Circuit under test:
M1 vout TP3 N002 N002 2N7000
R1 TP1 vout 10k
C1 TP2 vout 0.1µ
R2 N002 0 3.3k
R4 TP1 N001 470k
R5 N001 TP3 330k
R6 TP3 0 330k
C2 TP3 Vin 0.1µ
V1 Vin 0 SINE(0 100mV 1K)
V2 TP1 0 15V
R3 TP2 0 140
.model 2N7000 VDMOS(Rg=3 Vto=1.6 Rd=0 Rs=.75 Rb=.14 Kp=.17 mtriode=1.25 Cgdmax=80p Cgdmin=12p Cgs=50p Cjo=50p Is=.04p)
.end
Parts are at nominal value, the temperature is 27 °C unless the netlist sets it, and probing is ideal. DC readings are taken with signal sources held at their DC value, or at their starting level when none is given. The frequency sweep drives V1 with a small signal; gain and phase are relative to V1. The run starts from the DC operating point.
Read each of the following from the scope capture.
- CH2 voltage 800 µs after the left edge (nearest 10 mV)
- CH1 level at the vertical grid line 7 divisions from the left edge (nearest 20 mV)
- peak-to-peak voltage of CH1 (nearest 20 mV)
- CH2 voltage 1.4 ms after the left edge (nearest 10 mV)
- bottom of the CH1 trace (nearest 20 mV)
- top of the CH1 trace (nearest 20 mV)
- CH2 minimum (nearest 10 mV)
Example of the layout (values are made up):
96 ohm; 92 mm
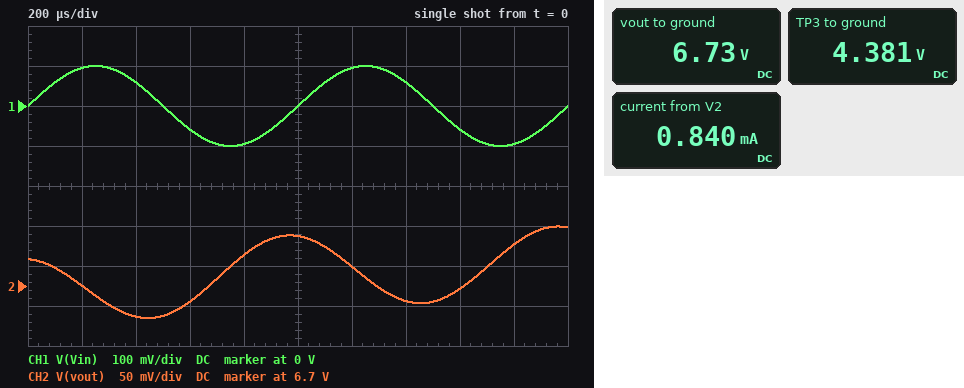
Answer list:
6.74 V; 60 mV; 200 mV; 6.68 V; -100 mV; 100 mV; 6.66 V
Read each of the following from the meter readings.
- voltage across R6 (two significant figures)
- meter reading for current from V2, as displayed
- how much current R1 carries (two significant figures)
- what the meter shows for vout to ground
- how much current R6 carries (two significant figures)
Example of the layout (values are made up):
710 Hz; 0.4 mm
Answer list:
4.4 V; 0.840 mA; 830 µA; 6.73 V; 13 µA
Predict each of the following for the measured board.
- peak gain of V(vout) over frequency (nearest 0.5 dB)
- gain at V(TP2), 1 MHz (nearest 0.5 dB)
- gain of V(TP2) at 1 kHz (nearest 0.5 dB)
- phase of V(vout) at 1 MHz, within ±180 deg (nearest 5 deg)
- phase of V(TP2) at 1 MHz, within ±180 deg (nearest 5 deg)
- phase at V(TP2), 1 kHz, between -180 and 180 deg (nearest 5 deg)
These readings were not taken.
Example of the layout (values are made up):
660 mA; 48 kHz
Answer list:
9.0 dB; -26.5 dB; -28.0 dB; 150 deg; 150 deg; -170 deg
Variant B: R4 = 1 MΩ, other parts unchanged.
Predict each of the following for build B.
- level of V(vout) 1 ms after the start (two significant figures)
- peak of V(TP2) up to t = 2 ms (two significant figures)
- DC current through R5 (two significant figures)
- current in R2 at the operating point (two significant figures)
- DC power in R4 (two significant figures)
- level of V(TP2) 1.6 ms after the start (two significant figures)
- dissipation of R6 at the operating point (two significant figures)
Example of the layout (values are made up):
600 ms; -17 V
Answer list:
11 V; 4.2 mV; 9.0 µA; 420 µA; 82 µW; 2.9 mV; 27 µW
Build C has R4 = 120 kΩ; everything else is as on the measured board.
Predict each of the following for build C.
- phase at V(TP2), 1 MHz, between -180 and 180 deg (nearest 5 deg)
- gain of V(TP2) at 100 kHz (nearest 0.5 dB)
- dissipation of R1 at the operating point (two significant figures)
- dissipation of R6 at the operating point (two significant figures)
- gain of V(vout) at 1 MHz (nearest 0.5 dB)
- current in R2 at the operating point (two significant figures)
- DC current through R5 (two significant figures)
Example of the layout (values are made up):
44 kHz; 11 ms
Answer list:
85 deg; -39.5 dB; 13 mW; 120 µW; -19.5 dB; 1.1 mA; 19 µA
